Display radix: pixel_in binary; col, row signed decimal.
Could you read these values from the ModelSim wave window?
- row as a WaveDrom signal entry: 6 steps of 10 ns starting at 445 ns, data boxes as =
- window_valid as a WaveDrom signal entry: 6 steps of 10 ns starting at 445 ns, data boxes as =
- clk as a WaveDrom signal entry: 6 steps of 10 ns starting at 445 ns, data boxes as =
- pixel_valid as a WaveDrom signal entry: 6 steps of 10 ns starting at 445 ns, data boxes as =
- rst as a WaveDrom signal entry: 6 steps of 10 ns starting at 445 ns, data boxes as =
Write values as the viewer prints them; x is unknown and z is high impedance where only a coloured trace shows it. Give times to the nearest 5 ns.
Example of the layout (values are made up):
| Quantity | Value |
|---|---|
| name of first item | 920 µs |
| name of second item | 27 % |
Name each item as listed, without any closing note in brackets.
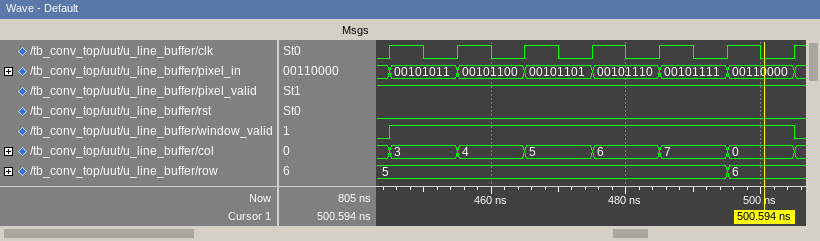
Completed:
| Quantity | Value |
|---|---|
| row as a WaveDrom signal entry: 6 steps of 10 ns starting at 445 ns, data boxes as = | {name: 'row', wave: '=....=', data: '5 6'} |
| window_valid as a WaveDrom signal entry: 6 steps of 10 ns starting at 445 ns, data boxes as = | {name: 'window_valid', wave: '1.....'} |
| clk as a WaveDrom signal entry: 6 steps of 10 ns starting at 445 ns, data boxes as = | {name: 'clk', wave: 'p.....'} |
| pixel_valid as a WaveDrom signal entry: 6 steps of 10 ns starting at 445 ns, data boxes as = | {name: 'pixel_valid', wave: '1.....'} |
| rst as a WaveDrom signal entry: 6 steps of 10 ns starting at 445 ns, data boxes as = | {name: 'rst', wave: '0.....'} |
